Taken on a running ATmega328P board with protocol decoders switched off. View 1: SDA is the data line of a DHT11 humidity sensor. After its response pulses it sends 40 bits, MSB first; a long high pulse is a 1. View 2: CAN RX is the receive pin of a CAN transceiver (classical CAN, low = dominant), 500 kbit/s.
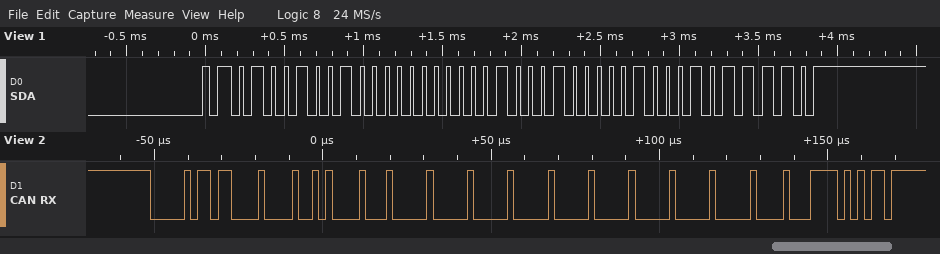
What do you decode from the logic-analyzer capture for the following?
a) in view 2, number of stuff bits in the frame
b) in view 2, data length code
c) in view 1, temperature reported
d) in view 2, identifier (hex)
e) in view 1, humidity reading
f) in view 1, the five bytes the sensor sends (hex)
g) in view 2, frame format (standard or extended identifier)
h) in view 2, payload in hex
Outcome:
10
8
17.4 °C
0x036
73 %
49 00 11 04 5E
standard
4A 11 00 00 00 00 00 00
